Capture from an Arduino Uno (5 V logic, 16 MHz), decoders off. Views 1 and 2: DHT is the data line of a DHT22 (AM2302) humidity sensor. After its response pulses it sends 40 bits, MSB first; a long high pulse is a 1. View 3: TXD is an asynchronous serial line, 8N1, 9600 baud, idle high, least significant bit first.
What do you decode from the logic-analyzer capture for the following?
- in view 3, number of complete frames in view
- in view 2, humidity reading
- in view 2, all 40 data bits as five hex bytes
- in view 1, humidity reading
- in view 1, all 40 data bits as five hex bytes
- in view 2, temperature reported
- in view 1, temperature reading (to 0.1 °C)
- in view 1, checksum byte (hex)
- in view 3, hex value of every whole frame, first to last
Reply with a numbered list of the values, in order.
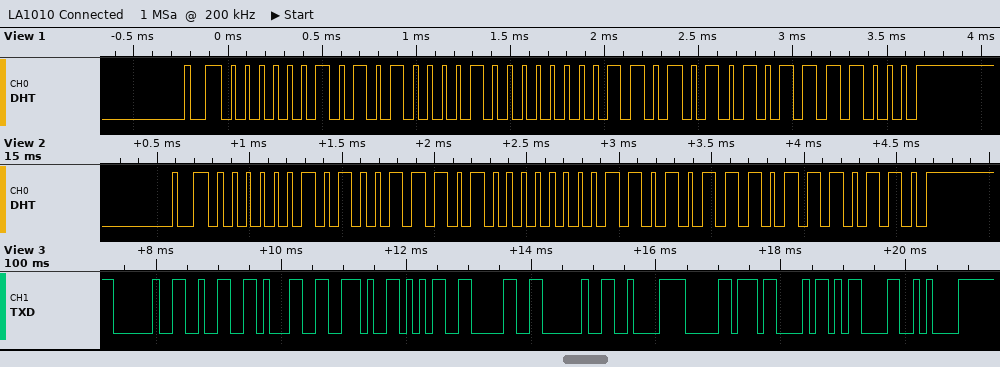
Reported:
1. 12
2. 66.9 %
3. 02 9D 00 D7 76
4. 67.3 %
5. 02 A1 00 D5 78
6. 21.5 °C
7. 21.3 °C
8. 0x78
9. 20 32 31 2E 35 30 20 C2 B0 43 0D 0A
